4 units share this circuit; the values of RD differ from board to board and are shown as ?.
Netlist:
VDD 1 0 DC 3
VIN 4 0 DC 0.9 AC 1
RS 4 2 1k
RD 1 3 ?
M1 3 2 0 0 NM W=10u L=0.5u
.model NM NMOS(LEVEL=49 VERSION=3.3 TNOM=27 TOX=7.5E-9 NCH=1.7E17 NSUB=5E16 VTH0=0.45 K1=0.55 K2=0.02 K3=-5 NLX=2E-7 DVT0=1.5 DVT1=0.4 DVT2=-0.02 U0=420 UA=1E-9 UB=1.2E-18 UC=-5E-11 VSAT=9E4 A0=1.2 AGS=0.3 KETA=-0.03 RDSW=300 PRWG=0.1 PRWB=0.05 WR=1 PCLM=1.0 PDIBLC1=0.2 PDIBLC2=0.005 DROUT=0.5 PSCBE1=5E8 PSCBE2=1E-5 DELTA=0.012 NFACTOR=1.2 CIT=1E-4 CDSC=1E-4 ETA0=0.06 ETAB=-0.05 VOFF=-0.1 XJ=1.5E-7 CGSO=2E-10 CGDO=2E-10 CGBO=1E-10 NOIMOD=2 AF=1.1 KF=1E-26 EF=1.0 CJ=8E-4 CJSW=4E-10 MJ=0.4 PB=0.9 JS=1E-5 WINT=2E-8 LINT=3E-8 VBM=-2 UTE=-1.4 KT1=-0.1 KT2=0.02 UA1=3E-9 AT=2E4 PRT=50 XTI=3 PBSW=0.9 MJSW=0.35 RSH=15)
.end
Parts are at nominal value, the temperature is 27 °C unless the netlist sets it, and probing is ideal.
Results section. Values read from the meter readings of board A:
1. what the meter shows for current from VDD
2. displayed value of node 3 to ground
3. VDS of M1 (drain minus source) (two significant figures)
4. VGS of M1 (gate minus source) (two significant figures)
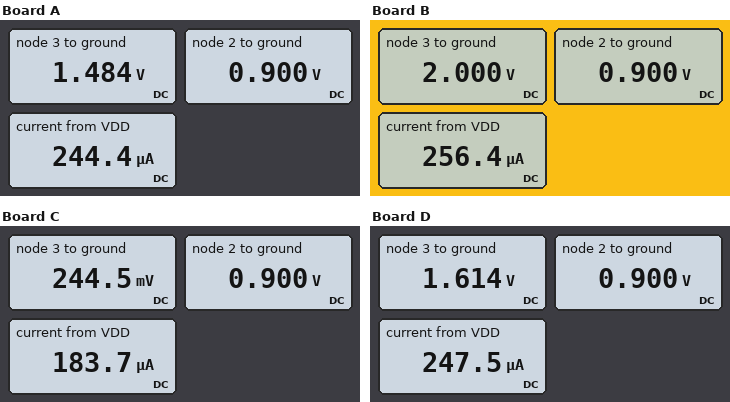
244.4 µA
1.484 V
1.5 V
900 mV
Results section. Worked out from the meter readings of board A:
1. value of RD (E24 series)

6.2 kΩ
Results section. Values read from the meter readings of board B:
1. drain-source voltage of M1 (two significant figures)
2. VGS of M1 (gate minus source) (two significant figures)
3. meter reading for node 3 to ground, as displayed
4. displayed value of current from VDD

2.0 V
900 mV
2.000 V
256.4 µA
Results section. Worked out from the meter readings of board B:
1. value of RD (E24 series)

3.9 kΩ
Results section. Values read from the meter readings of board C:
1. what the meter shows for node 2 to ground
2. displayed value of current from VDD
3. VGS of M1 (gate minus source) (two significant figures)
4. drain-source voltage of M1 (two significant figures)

0.900 V
183.7 µA
900 mV
240 mV
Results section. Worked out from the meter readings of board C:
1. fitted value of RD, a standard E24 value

15 kΩ
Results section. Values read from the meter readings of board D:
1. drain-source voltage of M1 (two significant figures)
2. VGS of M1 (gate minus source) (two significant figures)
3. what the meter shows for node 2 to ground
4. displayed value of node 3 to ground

1.6 V
900 mV
0.900 V
1.614 V
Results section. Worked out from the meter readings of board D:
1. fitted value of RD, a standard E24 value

5.6 kΩ
